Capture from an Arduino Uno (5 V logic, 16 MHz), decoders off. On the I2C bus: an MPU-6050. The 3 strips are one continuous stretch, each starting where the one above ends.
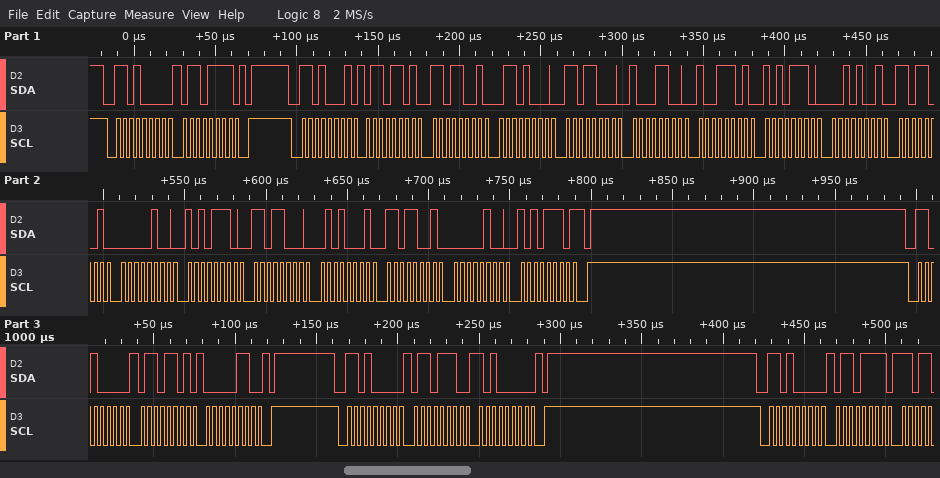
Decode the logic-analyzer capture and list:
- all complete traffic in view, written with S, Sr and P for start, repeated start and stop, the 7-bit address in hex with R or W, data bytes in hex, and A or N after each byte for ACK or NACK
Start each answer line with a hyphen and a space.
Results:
- S 68W A 6F A P S 68R A 6D A D9 A 68 A D8 A 8C A 9D A AE A 29 A D9 A 04 A AE A D8 A 51 A D9 A 04 A AE N P S 68W A 6D A 06 A P S 68W A 6E A A0 A P S 68W A 6F A
